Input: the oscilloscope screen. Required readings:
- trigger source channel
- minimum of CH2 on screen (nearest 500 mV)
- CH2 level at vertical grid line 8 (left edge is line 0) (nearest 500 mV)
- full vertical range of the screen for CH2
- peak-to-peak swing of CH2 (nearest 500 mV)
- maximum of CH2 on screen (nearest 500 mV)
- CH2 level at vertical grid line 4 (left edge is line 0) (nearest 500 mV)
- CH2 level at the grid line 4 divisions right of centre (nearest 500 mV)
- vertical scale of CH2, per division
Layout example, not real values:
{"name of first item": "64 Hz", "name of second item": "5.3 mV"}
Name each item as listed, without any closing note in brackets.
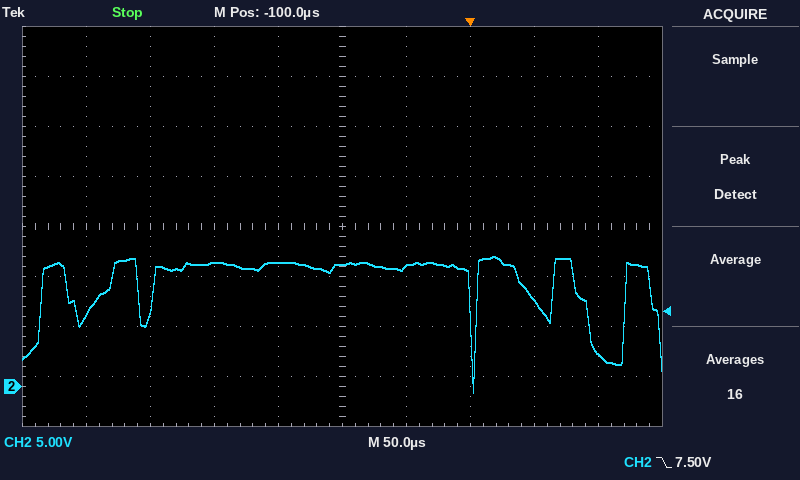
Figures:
{"trigger source channel": "CH2", "minimum of CH2 on screen": "-500 mV", "CH2 level at vertical grid line 8 (left edge is line 0)": "8.5 V", "full vertical range of the screen for CH2": "40 V", "peak-to-peak swing of CH2": "13.5 V", "maximum of CH2 on screen": "13.0 V", "CH2 level at vertical grid line 4 (left edge is line 0)": "12.5 V", "CH2 level at the grid line 4 divisions right of centre": "3.5 V", "vertical scale of CH2, per division": "5 V"}
